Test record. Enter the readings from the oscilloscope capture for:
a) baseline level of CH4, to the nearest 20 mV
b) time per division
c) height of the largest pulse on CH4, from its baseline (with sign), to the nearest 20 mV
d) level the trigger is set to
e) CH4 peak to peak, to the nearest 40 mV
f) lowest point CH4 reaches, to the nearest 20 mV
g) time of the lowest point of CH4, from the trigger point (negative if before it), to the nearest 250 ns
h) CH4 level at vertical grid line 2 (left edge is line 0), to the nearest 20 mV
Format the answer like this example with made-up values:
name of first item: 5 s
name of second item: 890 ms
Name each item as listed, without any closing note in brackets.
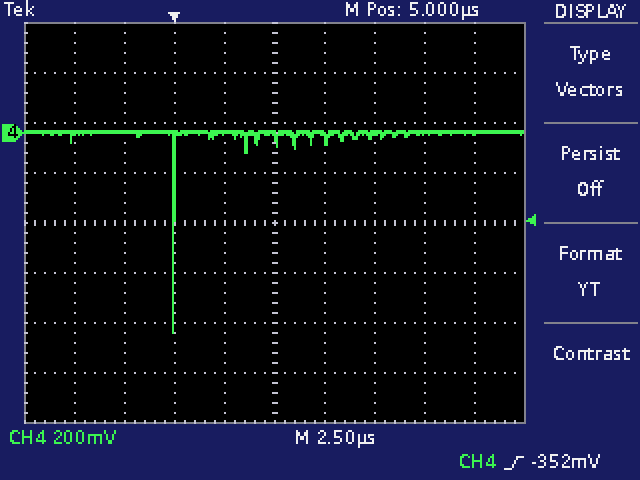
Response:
baseline level of CH4, to the nearest 20 mV: 0 mV
time per division: 2.5 µs
height of the largest pulse on CH4, from its baseline (with sign), to the nearest 20 mV: -800 mV
level the trigger is set to: -352 mV
CH4 peak to peak, to the nearest 40 mV: 800 mV
lowest point CH4 reaches, to the nearest 20 mV: -800 mV
time of the lowest point of CH4, from the trigger point (negative if before it), to the nearest 250 ns: 0.00 µs
CH4 level at vertical grid line 2 (left edge is line 0), to the nearest 20 mV: 0 mV
